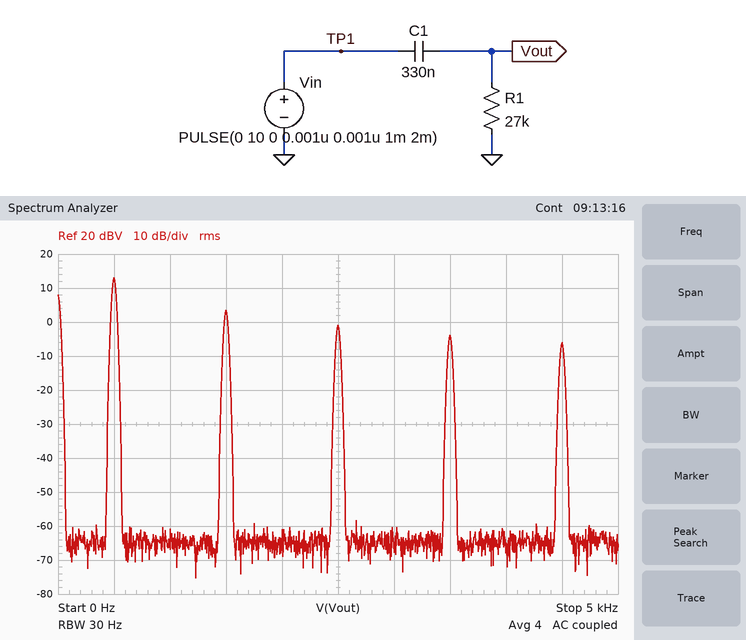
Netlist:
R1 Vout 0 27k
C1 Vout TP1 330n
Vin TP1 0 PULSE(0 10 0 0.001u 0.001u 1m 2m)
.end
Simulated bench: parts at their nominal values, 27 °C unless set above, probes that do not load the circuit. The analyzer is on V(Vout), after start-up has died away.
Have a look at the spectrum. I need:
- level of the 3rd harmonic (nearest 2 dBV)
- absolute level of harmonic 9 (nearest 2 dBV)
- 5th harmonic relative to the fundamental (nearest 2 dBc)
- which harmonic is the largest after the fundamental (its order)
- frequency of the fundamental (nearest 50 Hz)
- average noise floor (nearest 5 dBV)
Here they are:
4 dBV
-6 dBV
-14 dBc
3
500 Hz
-65 dBV
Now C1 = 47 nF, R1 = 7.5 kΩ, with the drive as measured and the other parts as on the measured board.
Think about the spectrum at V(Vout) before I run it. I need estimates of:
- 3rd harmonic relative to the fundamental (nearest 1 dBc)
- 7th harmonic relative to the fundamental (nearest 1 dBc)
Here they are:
-7 dBc
-14 dBc
